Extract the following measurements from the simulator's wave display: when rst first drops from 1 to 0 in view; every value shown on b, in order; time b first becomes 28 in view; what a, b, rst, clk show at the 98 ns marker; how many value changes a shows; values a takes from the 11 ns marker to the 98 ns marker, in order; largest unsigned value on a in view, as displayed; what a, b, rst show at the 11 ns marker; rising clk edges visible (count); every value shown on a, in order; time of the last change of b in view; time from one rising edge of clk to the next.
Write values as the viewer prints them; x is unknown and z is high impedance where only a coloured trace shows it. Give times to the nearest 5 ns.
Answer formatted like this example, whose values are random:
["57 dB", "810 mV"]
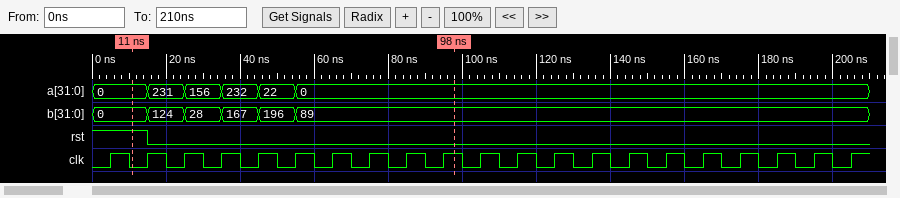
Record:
["15 ns", "0, 124, 28, 167, 196, 89", "25 ns", "a=0, b=89, rst=0, clk=1", "5", "0, 231, 156, 232, 22, 0", "232", "a=0, b=0, rst=1", "21", "0, 231, 156, 232, 22, 0", "55 ns", "10 ns"]
